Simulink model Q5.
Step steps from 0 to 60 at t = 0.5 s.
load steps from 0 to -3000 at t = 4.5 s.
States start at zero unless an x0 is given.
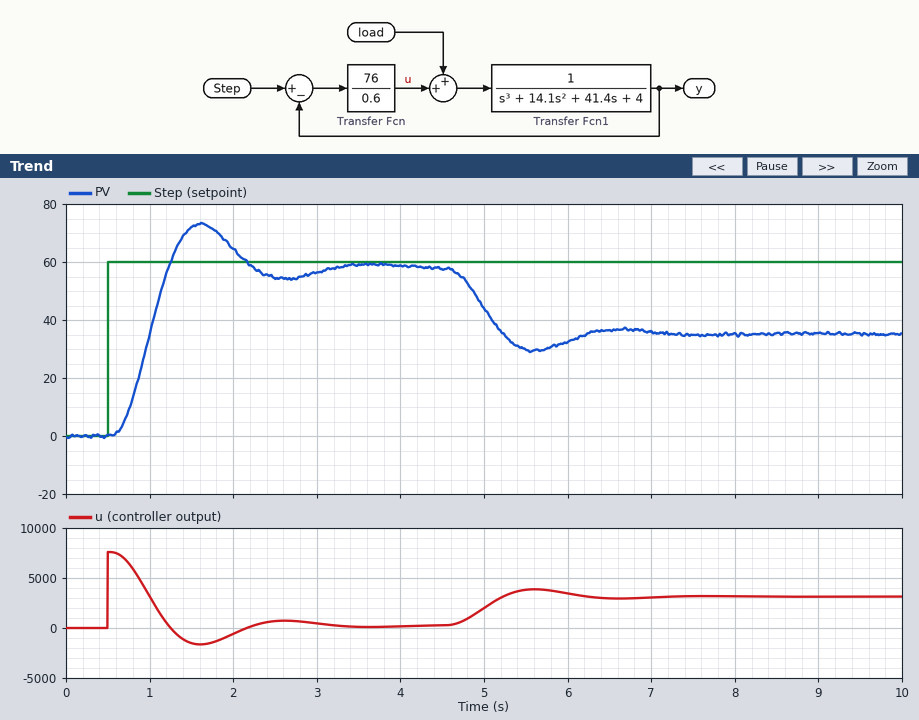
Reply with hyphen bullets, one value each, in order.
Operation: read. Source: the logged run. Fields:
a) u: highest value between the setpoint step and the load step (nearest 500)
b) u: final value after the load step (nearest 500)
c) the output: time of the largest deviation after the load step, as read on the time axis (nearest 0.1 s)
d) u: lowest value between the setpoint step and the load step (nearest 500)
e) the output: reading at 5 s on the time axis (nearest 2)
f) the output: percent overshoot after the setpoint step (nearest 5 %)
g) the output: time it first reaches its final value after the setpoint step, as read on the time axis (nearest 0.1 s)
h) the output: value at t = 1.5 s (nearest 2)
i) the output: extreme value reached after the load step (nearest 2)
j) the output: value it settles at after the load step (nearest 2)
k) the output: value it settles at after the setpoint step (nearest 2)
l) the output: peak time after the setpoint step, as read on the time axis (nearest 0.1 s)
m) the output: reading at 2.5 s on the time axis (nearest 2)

- 7500
- 3000
- 5.6 s
- -1500
- 44
- 25 %
- 1.2 s
- 72
- 30
- 36
- 58
- 1.6 s
- 54
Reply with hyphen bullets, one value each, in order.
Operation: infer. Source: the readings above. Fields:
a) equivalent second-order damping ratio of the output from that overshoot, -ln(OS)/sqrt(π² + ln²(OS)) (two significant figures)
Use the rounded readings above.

- 0.40
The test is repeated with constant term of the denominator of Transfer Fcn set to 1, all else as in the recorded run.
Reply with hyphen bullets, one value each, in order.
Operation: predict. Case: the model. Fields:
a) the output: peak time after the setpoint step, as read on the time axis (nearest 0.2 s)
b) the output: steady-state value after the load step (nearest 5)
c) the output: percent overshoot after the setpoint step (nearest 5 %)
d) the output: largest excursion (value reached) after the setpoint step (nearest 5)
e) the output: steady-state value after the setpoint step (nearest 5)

- 2.0 s
- 20
- 10 %
- 65
- 55
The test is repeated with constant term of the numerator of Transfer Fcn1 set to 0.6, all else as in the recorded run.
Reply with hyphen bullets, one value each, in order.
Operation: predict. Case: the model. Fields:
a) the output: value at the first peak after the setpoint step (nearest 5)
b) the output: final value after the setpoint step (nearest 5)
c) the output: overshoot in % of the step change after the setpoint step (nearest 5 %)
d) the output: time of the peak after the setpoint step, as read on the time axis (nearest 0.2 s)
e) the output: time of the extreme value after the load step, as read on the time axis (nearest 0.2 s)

- 65
- 55
- 10 %
- 2.0 s
- 6.0 s
